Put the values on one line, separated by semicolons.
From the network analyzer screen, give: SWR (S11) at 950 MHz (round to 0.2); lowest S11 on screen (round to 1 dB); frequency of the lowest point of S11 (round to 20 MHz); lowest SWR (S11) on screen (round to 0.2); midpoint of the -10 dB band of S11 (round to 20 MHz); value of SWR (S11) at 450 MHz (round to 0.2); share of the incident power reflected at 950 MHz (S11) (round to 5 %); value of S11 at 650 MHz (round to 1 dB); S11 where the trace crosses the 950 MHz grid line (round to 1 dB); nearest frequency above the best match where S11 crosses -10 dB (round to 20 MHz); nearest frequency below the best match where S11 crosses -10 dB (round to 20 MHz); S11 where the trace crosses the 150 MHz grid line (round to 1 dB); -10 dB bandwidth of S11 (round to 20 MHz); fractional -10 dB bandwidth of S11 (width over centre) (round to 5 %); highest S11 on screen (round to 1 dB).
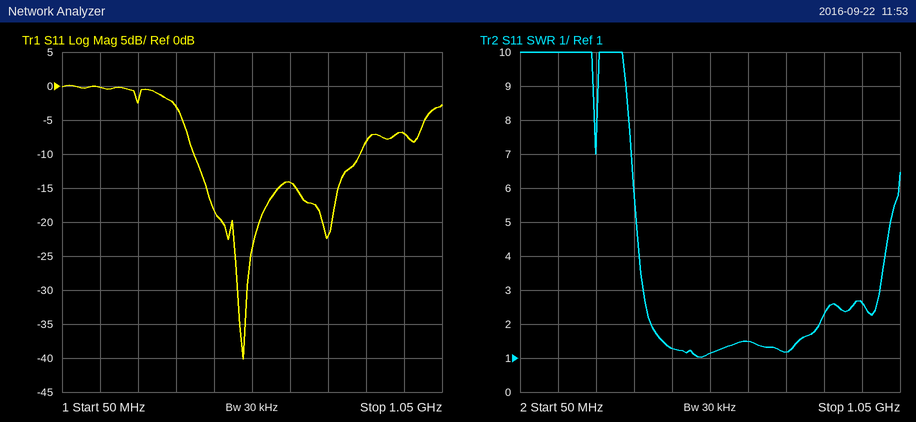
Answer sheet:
2.6; -40 dB; 520 MHz; 1.0; 620 MHz; 1.2; 20 %; -14 dB; -7 dB; 840 MHz; 400 MHz; 0 dB; 440 MHz; 70 %; 0 dB
